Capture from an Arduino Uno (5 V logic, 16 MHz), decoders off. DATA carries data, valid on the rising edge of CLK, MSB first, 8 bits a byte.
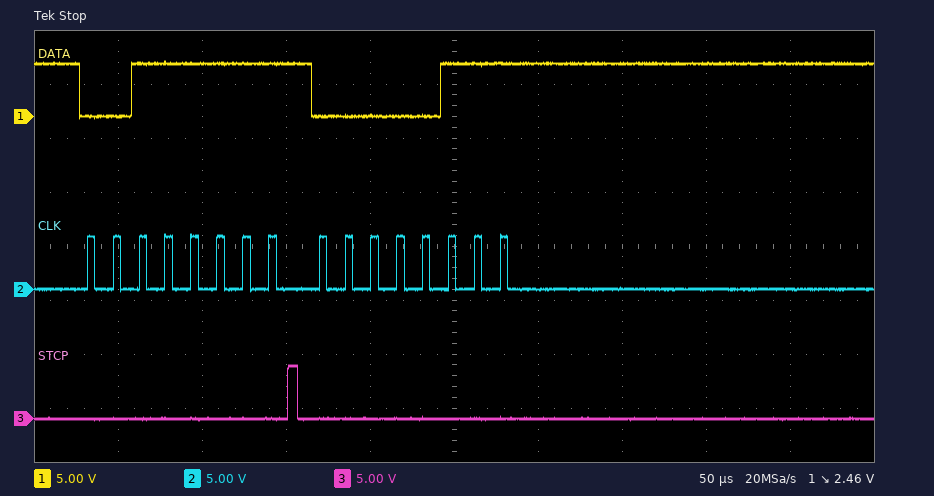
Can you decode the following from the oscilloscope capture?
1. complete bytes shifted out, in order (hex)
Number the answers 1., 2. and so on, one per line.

1. 0x3F 0x07
